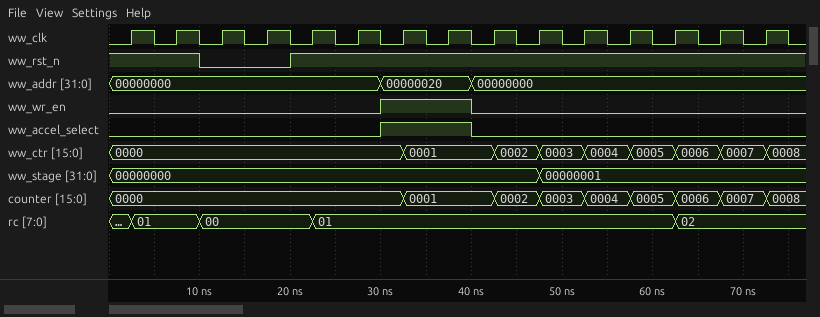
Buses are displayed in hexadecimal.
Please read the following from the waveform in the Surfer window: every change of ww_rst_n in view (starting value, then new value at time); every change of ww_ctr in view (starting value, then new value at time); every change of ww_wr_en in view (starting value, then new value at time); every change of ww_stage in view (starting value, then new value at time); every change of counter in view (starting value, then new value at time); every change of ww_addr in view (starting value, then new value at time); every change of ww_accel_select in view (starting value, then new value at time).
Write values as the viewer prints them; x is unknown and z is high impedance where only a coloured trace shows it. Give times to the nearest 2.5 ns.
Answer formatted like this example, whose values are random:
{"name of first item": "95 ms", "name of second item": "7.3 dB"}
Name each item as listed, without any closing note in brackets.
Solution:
{"every change of ww_rst_n in view": "1, 0 at 10 ns, 1 at 20 ns", "every change of ww_ctr in view": "0000, 0001 at 32.5 ns, 0002 at 42.5 ns, 0003 at 47.5 ns, 0004 at 52.5 ns, 0005 at 57.5 ns, 0006 at 62.5 ns, 0007 at 67.5 ns, 0008 at 72.5 ns", "every change of ww_wr_en in view": "0, 1 at 30 ns, 0 at 40 ns", "every change of ww_stage in view": "00000000, 00000001 at 47.5 ns", "every change of counter in view": "0000, 0001 at 32.5 ns, 0002 at 42.5 ns, 0003 at 47.5 ns, 0004 at 52.5 ns, 0005 at 57.5 ns, 0006 at 62.5 ns, 0007 at 67.5 ns, 0008 at 72.5 ns", "every change of ww_addr in view": "00000000, 00000020 at 30 ns, 00000000 at 40 ns", "every change of ww_accel_select in view": "0, 1 at 30 ns, 0 at 40 ns"}
